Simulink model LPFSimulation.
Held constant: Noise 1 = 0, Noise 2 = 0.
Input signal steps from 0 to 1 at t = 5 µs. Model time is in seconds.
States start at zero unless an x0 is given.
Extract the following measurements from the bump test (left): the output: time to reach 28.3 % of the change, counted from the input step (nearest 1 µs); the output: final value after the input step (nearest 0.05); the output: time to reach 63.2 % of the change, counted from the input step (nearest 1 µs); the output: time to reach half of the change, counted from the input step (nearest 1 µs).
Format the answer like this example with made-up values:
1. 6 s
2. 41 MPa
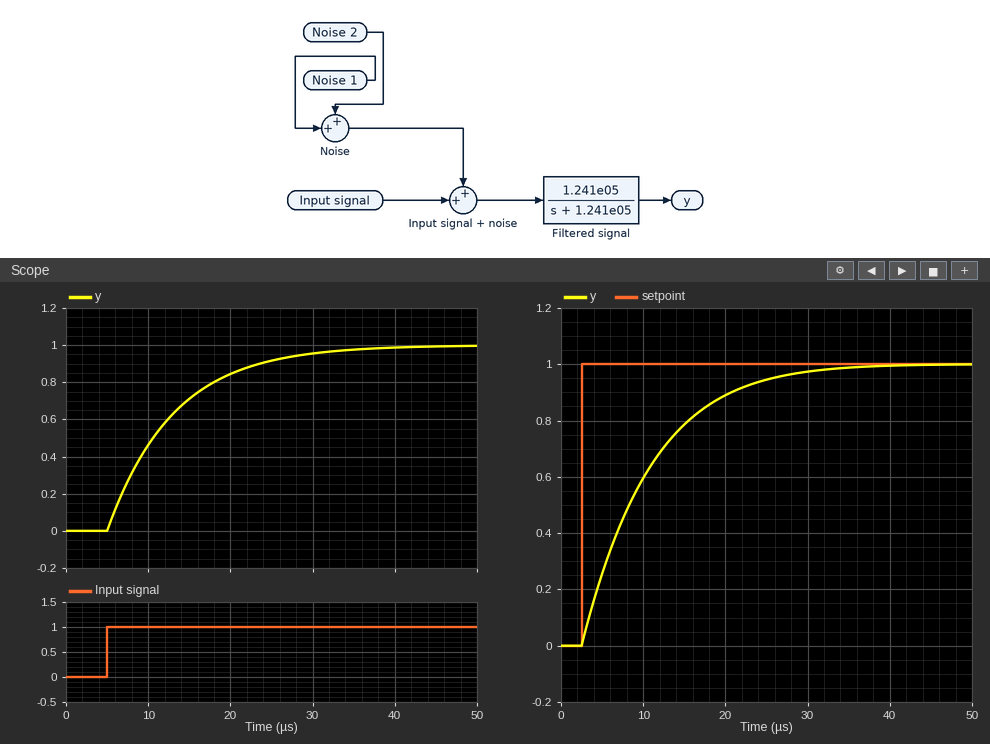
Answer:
1. 3 µs
2. 1.00
3. 8 µs
4. 6 µs
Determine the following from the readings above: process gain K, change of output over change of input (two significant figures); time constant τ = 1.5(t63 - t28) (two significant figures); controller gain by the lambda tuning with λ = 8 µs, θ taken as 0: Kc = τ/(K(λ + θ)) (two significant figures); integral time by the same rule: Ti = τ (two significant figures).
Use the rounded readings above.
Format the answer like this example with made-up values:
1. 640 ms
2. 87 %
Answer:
1. 1.0
2. 7.5 µs
3. 0.94
4. 7.5 µs
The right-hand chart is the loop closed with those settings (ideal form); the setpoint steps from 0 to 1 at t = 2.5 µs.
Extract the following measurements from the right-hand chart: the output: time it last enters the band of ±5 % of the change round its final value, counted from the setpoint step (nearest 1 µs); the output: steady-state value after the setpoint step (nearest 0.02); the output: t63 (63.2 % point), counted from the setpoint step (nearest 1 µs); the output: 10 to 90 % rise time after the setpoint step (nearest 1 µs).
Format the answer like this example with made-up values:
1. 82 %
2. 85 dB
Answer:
1. 23 µs
2. 1.00
3. 8 µs
4. 17 µs
